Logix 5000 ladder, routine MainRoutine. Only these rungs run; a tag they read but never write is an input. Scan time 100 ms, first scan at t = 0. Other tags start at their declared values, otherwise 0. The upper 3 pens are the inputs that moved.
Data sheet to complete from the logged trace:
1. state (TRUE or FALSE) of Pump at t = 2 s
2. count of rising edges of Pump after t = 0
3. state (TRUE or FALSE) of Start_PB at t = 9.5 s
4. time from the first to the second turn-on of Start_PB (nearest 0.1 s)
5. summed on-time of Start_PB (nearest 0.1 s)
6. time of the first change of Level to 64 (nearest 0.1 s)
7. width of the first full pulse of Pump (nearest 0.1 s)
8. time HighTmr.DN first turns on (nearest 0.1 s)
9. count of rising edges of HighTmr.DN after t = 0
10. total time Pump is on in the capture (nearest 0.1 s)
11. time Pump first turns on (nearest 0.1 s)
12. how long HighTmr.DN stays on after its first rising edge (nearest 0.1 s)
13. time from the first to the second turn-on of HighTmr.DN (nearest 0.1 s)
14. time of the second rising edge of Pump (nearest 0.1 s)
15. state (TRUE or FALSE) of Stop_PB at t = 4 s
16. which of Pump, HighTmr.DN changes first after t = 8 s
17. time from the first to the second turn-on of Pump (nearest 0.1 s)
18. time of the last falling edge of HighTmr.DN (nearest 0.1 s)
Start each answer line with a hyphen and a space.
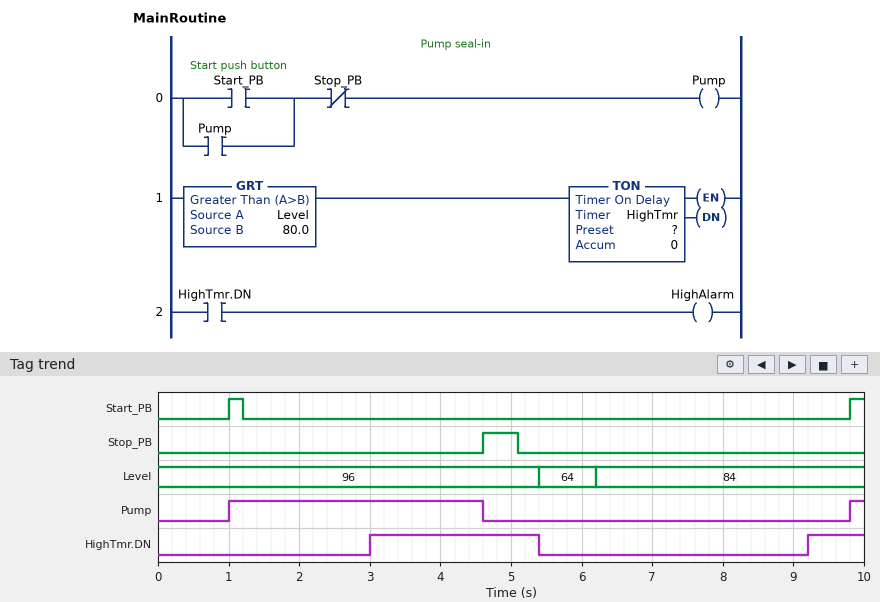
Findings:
- TRUE
- 2
- FALSE
- 8.8 s
- 0.4 s
- 5.4 s
- 3.6 s
- 3.0 s
- 2
- 3.8 s
- 1.0 s
- 2.4 s
- 6.2 s
- 9.8 s
- FALSE
- HighTmr.DN
- 8.8 s
- 5.4 s
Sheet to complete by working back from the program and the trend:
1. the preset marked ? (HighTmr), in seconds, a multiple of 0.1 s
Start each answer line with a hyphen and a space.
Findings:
- 3.0 s
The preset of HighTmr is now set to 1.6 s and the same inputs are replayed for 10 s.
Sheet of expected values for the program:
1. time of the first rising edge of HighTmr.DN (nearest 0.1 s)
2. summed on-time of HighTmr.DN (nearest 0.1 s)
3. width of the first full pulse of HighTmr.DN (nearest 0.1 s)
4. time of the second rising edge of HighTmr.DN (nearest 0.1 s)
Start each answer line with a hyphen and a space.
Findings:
- 1.6 s
- 6.0 s
- 3.8 s
- 7.8 s
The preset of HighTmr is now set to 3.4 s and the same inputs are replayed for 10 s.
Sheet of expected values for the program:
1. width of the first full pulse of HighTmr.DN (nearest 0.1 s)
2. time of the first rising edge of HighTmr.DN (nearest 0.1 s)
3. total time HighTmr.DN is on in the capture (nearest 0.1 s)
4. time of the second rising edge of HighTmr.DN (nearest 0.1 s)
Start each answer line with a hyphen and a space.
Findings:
- 2.0 s
- 3.4 s
- 2.4 s
- 9.6 s
